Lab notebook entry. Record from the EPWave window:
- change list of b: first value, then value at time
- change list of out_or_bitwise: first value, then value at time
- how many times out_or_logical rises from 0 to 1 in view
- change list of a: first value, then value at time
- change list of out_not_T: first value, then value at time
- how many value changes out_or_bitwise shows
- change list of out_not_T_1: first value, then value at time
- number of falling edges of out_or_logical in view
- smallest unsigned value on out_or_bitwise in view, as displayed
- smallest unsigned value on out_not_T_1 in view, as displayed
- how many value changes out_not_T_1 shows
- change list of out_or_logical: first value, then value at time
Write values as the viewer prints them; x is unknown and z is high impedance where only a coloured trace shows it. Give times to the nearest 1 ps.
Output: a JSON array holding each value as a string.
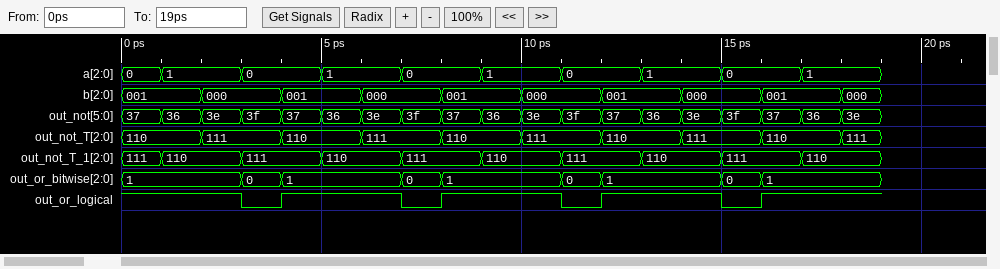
["001, 000 at 2 ps, 001 at 4 ps, 000 at 6 ps, 001 at 8 ps, 000 at 10 ps, 001 at 12 ps, 000 at 14 ps, 001 at 16 ps, 000 at 18 ps", "1, 0 at 3 ps, 1 at 4 ps, 0 at 7 ps, 1 at 8 ps, 0 at 11 ps, 1 at 12 ps, 0 at 15 ps, 1 at 16 ps", "4", "0, 1 at 1 ps, 0 at 3 ps, 1 at 5 ps, 0 at 7 ps, 1 at 9 ps, 0 at 11 ps, 1 at 13 ps, 0 at 15 ps, 1 at 17 ps", "110, 111 at 2 ps, 110 at 4 ps, 111 at 6 ps, 110 at 8 ps, 111 at 10 ps, 110 at 12 ps, 111 at 14 ps, 110 at 16 ps, 111 at 18 ps", "8", "111, 110 at 1 ps, 111 at 3 ps, 110 at 5 ps, 111 at 7 ps, 110 at 9 ps, 111 at 11 ps, 110 at 13 ps, 111 at 15 ps, 110 at 17 ps", "4", "0", "110", "9", "1, 0 at 3 ps, 1 at 4 ps, 0 at 7 ps, 1 at 8 ps, 0 at 11 ps, 1 at 12 ps, 0 at 15 ps, 1 at 16 ps"]
